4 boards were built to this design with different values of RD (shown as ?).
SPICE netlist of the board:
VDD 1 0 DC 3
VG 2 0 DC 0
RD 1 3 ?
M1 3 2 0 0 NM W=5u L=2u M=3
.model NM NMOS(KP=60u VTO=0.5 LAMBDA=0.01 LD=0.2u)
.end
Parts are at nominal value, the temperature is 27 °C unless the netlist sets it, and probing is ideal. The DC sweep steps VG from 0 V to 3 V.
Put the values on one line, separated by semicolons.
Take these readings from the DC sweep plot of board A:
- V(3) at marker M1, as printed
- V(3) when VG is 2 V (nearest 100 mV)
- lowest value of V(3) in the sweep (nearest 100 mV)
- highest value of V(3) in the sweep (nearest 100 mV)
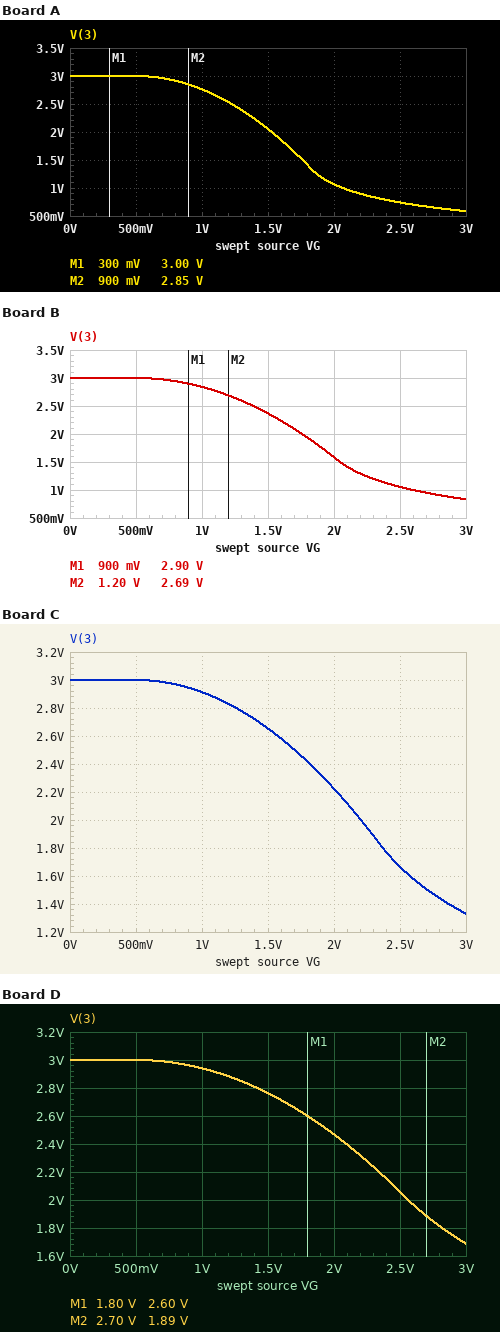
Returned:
3.00 V; 1.1 V; 600 mV; 3.0 V
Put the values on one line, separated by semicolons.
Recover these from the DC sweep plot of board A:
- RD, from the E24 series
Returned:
3.3 kΩ
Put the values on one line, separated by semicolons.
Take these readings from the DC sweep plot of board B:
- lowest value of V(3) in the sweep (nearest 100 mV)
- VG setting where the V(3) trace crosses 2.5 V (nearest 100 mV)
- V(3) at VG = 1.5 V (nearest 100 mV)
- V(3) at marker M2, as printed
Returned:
800 mV; 1.4 V; 2.4 V; 2.69 V
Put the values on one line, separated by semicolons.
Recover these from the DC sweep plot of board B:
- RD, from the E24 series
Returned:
2.2 kΩ
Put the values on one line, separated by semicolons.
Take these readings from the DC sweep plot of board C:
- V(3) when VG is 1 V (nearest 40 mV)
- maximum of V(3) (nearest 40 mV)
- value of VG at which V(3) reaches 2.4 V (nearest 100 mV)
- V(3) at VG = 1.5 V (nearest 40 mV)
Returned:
2.92 V; 3.00 V; 1.8 V; 2.64 V
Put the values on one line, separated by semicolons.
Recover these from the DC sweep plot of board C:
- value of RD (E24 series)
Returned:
1.2 kΩ
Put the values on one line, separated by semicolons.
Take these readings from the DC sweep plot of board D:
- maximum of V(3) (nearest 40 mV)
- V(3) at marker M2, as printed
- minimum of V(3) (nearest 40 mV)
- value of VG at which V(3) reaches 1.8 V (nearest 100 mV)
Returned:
3.00 V; 1.89 V; 1.68 V; 2.8 V
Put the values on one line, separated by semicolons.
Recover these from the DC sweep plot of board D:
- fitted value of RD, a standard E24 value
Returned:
820 Ω
